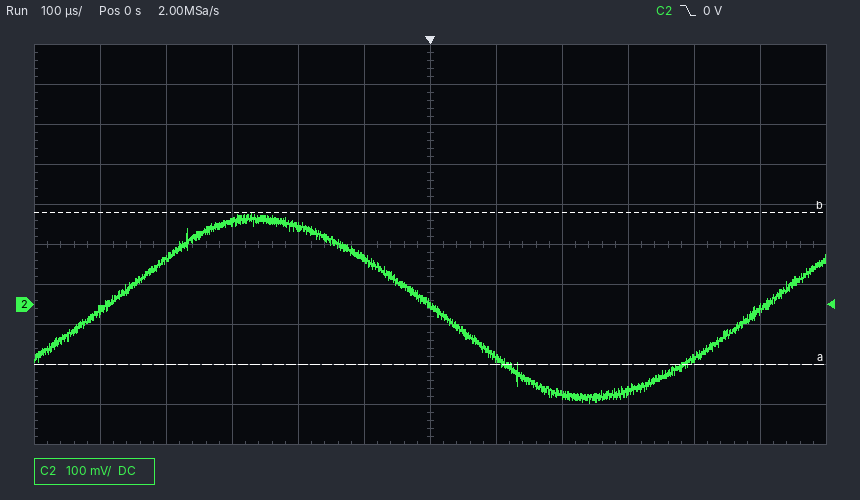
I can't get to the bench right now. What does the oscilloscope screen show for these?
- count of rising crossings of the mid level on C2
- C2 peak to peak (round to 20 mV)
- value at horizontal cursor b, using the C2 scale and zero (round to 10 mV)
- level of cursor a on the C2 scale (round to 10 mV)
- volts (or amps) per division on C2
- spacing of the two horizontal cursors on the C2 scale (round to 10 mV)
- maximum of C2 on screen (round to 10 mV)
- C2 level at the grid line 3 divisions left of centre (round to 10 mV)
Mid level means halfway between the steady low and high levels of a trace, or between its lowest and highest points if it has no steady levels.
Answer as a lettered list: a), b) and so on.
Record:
a) 2
b) 480 mV
c) 230 mV
d) -150 mV
e) 100 mV
f) 380 mV
g) 230 mV
h) 210 mV
